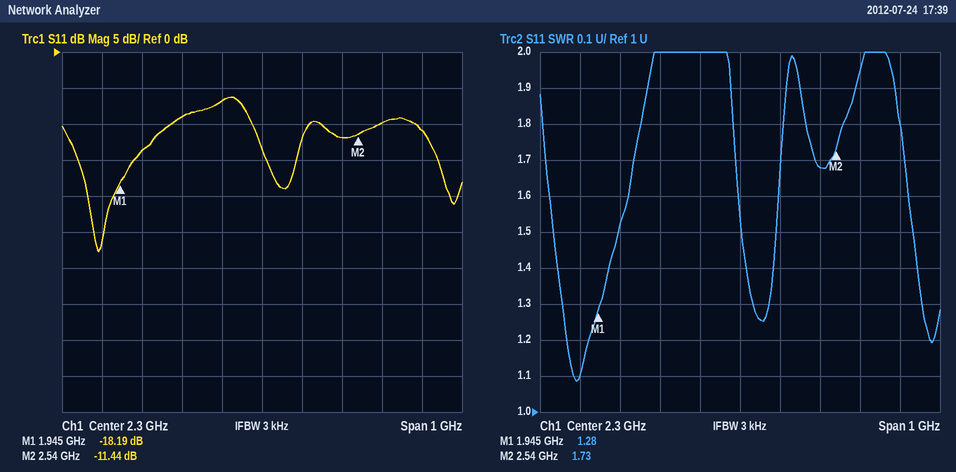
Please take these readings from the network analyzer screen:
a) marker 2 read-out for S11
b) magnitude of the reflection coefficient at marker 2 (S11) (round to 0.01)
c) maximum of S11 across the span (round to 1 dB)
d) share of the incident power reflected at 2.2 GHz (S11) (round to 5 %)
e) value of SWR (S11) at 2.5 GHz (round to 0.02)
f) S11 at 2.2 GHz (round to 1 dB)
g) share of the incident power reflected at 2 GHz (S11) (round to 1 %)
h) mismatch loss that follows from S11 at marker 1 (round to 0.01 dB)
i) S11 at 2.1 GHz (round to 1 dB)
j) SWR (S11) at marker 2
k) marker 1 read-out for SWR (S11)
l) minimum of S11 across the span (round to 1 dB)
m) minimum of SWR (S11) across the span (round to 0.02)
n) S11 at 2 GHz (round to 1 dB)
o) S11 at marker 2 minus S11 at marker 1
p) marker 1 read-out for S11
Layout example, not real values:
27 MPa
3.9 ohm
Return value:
-11.44 dB
0.27
-6 dB
20 %
1.68
-7 dB
4 %
0.07 dB
-9 dB
1.73
1.28
-28 dB
1.08
-14 dB
6.75 dB
-18.19 dB
